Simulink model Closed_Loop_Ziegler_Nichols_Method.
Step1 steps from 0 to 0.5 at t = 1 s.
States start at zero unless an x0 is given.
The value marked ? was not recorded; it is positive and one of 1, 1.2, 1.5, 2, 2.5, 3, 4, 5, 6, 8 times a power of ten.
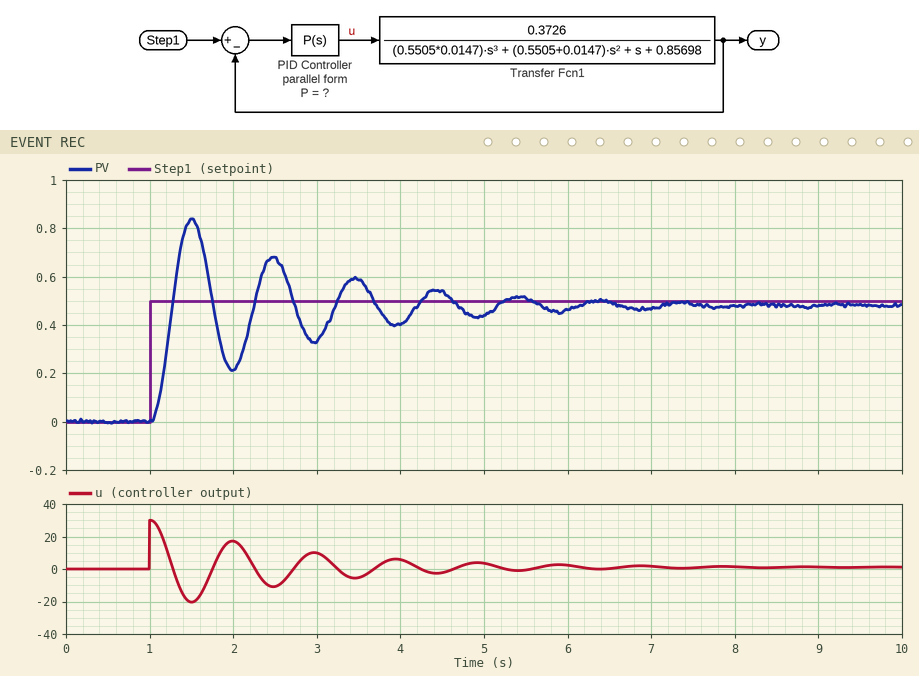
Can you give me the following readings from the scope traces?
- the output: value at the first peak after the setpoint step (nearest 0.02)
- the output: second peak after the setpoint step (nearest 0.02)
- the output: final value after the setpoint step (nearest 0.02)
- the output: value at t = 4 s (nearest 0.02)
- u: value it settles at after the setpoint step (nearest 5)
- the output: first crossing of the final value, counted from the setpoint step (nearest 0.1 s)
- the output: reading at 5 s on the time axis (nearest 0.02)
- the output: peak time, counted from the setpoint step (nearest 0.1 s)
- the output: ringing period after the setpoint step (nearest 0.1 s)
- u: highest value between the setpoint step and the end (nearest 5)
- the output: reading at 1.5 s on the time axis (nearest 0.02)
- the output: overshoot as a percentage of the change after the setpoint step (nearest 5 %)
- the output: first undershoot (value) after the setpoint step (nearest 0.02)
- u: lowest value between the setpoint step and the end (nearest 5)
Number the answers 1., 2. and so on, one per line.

1. 0.84
2. 0.68
3. 0.48
4. 0.40
5. 0
6. 0.3 s
7. 0.44
8. 0.5 s
9. 1.0 s
10. 30
11. 0.84
12. 75 %
13. 0.22
14. -20
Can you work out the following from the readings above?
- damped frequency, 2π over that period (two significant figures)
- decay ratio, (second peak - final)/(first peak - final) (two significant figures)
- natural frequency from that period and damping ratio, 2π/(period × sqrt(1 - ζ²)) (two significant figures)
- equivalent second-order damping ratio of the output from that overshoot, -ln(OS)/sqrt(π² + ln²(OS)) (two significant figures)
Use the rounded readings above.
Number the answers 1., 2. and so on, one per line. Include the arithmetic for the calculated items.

1. 2π / 1 = 6.3 rad/s
2. (0.68 - 0.48) / (0.84 - 0.48) = 0.56
3. 2π / (1 × sqrt(1 - 0.091²)) = 6.3 rad/s
4. ln(0.75) = -0.288; 0.288 / sqrt(9.870 + 0.083) = 0.091
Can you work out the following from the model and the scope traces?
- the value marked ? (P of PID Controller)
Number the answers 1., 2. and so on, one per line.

1. 60
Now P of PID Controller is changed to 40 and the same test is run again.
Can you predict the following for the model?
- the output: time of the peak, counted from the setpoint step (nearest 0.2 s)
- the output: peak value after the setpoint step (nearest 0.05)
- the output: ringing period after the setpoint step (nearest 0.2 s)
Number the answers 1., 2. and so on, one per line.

1. 0.6 s
2. 0.80
3. 1.2 s
